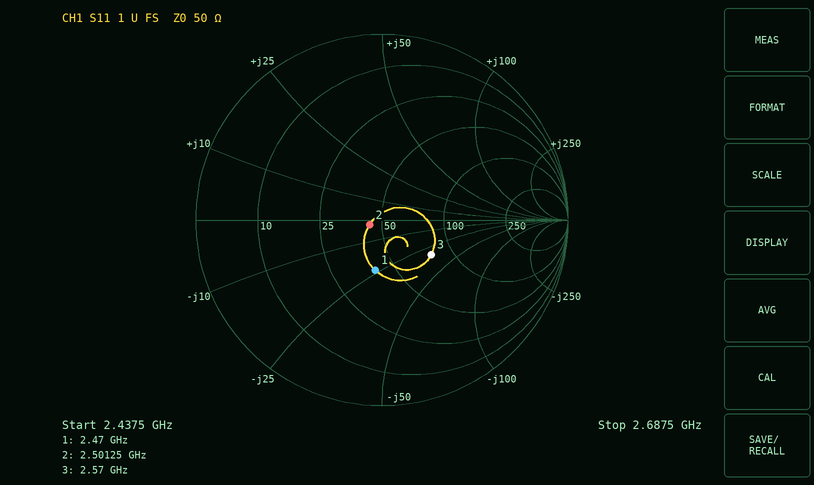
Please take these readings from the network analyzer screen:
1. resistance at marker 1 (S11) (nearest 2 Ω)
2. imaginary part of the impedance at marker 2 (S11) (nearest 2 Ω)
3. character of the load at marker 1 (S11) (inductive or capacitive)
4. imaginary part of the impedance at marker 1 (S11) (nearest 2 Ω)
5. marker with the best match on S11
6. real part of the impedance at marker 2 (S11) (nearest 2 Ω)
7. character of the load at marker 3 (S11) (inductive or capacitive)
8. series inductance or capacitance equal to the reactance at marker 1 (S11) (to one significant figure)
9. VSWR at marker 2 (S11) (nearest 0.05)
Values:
40 Ω
-2 Ω
capacitive
-24 Ω
marker 2
44 Ω
capacitive
3 pF
1.15
